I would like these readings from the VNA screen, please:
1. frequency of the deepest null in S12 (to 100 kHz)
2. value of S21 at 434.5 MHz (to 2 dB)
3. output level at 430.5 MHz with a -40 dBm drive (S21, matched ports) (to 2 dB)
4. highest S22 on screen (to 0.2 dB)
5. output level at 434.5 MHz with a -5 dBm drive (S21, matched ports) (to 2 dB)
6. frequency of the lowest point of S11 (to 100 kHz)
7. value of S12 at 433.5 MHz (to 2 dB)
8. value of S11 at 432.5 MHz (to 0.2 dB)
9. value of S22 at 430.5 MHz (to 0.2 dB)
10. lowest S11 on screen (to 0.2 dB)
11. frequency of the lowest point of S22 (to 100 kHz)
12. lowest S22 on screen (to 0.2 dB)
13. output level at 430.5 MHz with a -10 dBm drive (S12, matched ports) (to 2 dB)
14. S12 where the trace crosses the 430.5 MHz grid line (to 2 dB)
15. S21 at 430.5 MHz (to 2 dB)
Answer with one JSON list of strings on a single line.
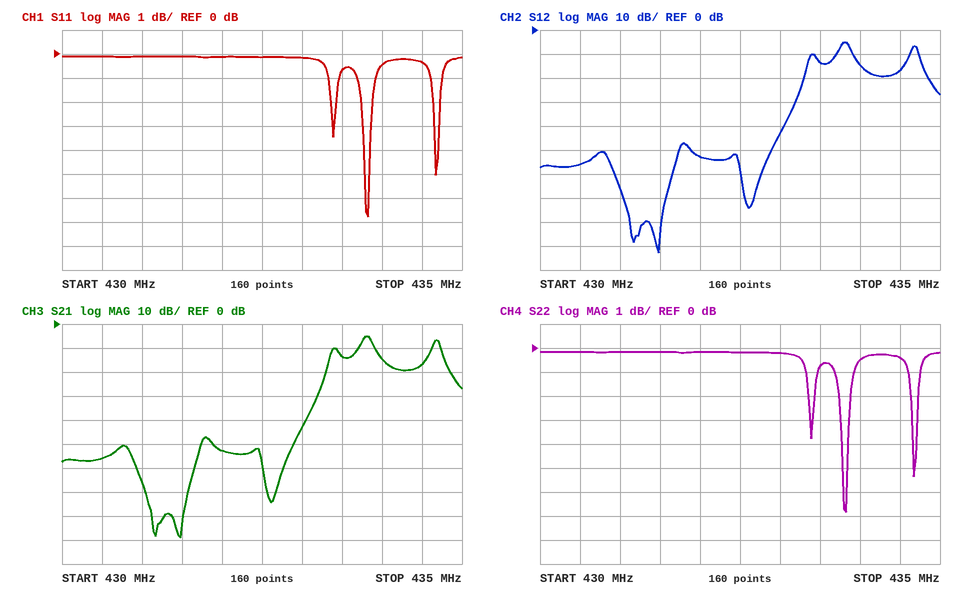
["431.5 MHz", "-16 dB", "-96 dBm", "-0.2 dB", "-22 dBm", "433.8 MHz", "-14 dB", "-0.2 dB", "-0.2 dB", "-6.8 dB", "433.8 MHz", "-6.8 dB", "-66 dBm", "-56 dB", "-56 dB"]
